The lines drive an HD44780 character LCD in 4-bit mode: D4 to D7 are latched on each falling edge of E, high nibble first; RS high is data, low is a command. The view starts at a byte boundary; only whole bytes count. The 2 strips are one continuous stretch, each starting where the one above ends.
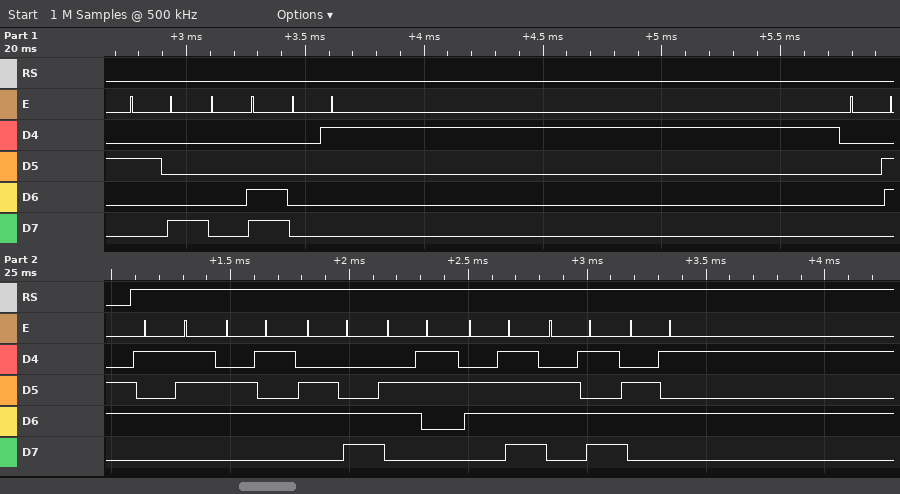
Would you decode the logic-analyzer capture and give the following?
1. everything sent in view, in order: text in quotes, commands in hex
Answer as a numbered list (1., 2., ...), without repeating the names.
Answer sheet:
1. 0x28 0x0C 0x01 0x06 "Welcome"
